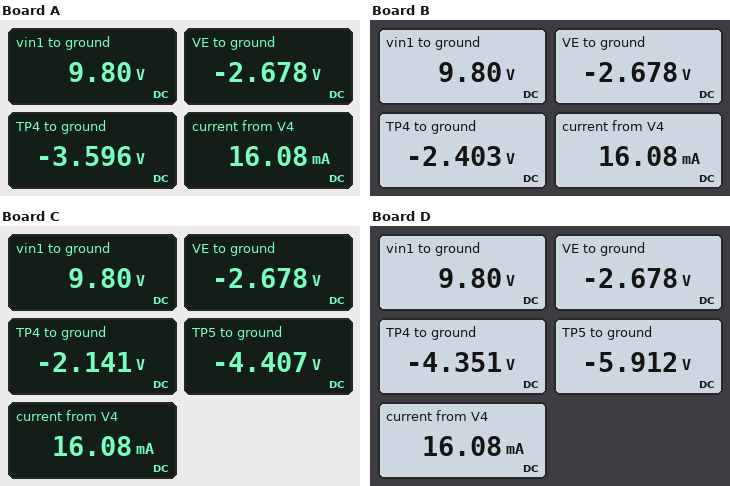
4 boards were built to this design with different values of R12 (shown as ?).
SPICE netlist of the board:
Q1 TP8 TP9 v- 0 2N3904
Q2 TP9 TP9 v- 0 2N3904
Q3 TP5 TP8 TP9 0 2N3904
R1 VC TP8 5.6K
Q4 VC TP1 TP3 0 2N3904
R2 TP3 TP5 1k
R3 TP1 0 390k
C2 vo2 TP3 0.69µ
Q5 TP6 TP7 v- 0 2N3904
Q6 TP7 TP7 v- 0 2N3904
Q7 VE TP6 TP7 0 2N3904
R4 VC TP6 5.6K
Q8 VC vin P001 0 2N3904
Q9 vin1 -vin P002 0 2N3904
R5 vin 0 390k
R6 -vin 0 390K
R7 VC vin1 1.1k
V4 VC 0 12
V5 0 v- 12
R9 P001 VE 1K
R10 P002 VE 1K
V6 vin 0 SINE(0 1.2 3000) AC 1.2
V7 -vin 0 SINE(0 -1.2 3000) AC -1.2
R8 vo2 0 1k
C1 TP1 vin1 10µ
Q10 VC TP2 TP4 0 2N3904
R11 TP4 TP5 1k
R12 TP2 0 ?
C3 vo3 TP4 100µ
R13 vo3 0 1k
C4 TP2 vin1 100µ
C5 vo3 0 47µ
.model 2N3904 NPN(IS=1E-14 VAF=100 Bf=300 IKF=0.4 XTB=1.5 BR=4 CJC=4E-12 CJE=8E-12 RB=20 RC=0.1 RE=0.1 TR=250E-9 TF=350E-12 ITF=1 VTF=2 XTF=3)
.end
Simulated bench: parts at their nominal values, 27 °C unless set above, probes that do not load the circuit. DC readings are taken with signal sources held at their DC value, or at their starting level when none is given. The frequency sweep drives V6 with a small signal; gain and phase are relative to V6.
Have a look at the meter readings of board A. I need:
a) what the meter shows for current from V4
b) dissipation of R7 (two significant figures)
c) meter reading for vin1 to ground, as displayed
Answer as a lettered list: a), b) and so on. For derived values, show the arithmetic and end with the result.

a) 16.08 mA
b) (12 V - 9.8 V)^2 / 1.1 kΩ = 4.4 mW
c) 9.80 V
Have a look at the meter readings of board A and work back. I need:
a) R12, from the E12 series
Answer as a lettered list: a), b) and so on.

a) 560 kΩ
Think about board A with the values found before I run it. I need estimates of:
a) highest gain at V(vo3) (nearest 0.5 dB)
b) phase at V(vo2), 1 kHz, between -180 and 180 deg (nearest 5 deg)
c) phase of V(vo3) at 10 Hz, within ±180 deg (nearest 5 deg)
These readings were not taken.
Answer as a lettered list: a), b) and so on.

a) -2.0 dB
b) 10 deg
c) 5 deg
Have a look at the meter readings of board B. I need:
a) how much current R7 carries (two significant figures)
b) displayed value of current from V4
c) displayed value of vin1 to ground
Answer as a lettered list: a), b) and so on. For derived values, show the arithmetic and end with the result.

a) (12 V - 9.8 V) / 1.1 kΩ = 2.0 mA
b) 16.08 mA
c) 9.80 V
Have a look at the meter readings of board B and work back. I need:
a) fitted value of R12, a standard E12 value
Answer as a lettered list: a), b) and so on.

a) 270 kΩ
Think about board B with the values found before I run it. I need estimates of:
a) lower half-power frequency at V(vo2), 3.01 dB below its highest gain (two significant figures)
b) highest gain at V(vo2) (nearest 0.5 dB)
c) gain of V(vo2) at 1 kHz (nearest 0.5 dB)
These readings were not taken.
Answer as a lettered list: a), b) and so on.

a) 160 Hz
b) -1.0 dB
c) -1.0 dB
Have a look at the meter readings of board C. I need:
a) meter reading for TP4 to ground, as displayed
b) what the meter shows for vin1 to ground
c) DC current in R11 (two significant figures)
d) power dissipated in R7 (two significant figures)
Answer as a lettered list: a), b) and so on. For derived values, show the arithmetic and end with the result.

a) -2.141 V
b) 9.80 V
c) (-2.141 V - (-4.407 V)) / 1 kΩ = 2.3 mA
d) (12 V - 9.8 V)^2 / 1.1 kΩ = 4.4 mW
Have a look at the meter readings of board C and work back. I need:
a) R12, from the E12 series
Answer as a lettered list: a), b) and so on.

a) 220 kΩ
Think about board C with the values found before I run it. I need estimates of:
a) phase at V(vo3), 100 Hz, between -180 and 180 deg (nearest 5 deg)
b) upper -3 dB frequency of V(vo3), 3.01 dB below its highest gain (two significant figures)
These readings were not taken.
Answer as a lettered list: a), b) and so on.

a) -15 deg
b) 340 Hz
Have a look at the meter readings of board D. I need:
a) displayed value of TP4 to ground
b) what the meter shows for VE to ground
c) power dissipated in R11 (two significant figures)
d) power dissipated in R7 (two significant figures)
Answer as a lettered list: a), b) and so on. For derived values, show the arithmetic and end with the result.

a) -4.351 V
b) -2.678 V
c) (-4.351 V - (-5.912 V))^2 / 1 kΩ = 2.4 mW
d) (12 V - 9.8 V)^2 / 1.1 kΩ = 4.4 mW
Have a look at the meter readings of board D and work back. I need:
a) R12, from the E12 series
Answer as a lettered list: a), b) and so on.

a) 820 kΩ
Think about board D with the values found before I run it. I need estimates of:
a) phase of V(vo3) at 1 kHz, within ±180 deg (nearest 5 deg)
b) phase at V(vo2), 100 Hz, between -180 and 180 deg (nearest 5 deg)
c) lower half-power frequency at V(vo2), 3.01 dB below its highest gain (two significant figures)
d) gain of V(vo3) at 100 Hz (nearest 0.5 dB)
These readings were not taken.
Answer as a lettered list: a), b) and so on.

a) -75 deg
b) 65 deg
c) 180 Hz
d) -2.5 dB
